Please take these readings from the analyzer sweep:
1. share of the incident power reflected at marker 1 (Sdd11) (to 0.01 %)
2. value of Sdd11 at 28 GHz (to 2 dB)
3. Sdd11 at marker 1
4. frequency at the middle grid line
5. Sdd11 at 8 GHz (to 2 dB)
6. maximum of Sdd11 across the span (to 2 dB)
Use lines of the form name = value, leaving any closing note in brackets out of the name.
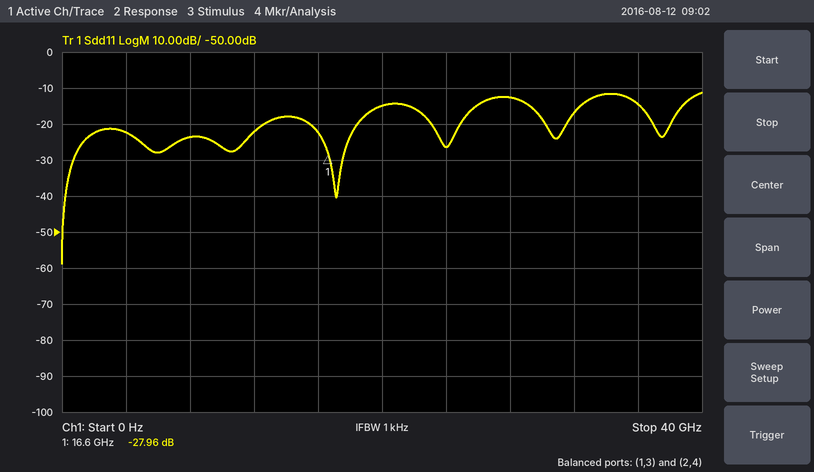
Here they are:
share of the incident power reflected at marker 1 (Sdd11) = 0.16 %
value of Sdd11 at 28 GHz = -12 dB
Sdd11 at marker 1 = -27.96 dB
frequency at the middle grid line = 20 GHz
Sdd11 at 8 GHz = -24 dB
maximum of Sdd11 across the span = -12 dB
